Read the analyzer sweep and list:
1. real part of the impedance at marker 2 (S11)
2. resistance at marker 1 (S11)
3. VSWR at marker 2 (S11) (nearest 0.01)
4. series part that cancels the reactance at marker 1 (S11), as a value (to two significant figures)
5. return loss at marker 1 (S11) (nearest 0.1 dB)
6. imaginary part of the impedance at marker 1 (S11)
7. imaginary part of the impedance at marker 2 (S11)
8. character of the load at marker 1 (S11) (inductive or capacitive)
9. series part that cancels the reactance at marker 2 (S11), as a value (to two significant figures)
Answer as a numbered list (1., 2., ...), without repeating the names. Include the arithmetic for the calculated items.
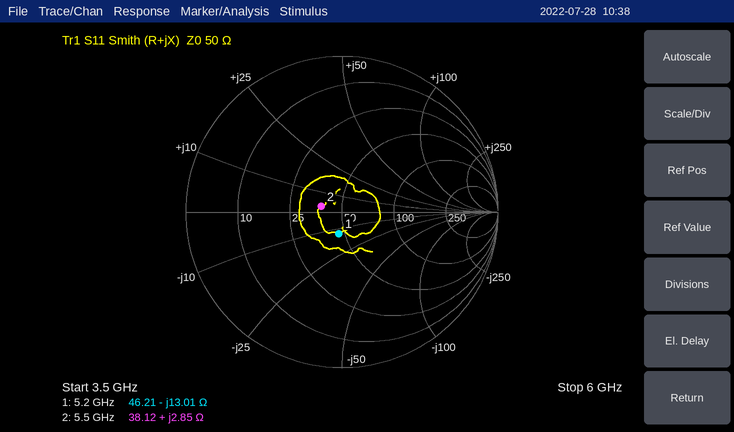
1. 38.12 Ω
2. 46.21 Ω
3. 1.32
4. L = 13.01 Ω/(2π × 5.2 GHz) ≈ 398 pH, so 400 pH to two significant figures
5. 17.1 dB
6. -13.01 Ω
7. +2.85 Ω
8. capacitive
9. C = 1/(2π × 5.5 GHz × 2.85 Ω) ≈ 10 pF
